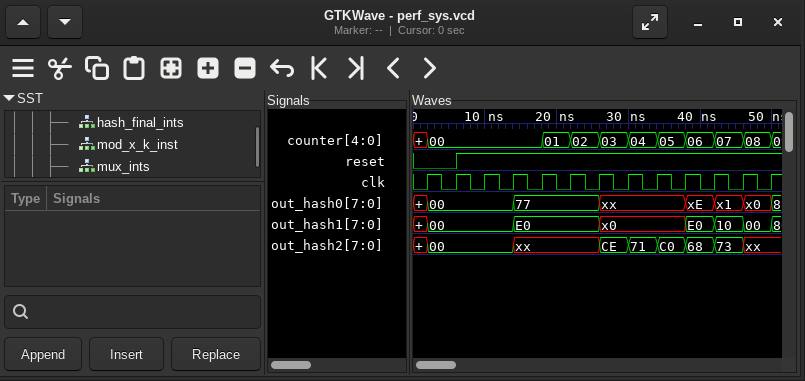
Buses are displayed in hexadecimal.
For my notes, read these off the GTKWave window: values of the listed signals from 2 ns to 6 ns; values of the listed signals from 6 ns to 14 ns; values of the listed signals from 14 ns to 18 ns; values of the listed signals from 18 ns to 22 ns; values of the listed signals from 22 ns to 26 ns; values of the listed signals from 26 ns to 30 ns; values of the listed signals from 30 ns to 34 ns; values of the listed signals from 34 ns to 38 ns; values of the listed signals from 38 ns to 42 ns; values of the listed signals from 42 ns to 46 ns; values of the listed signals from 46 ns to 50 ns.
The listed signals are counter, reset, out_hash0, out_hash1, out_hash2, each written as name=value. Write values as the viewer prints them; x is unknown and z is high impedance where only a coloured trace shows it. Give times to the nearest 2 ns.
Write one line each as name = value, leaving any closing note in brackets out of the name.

values of the listed signals from 2 ns to 6 ns = counter=00, reset=0, out_hash0=00, out_hash1=00, out_hash2=00
values of the listed signals from 6 ns to 14 ns = counter=00, reset=1, out_hash0=00, out_hash1=00, out_hash2=00
values of the listed signals from 14 ns to 18 ns = counter=00, reset=1, out_hash0=77, out_hash1=E0, out_hash2=xx
values of the listed signals from 18 ns to 22 ns = counter=01, reset=1, out_hash0=77, out_hash1=E0, out_hash2=xx
values of the listed signals from 22 ns to 26 ns = counter=02, reset=1, out_hash0=77, out_hash1=E0, out_hash2=xx
values of the listed signals from 26 ns to 30 ns = counter=03, reset=1, out_hash0=xx, out_hash1=x0, out_hash2=CE
values of the listed signals from 30 ns to 34 ns = counter=04, reset=1, out_hash0=xx, out_hash1=x0, out_hash2=71
values of the listed signals from 34 ns to 38 ns = counter=05, reset=1, out_hash0=xx, out_hash1=x0, out_hash2=C0
values of the listed signals from 38 ns to 42 ns = counter=06, reset=1, out_hash0=xE, out_hash1=E0, out_hash2=68
values of the listed signals from 42 ns to 46 ns = counter=07, reset=1, out_hash0=x1, out_hash1=10, out_hash2=73
values of the listed signals from 46 ns to 50 ns = counter=08, reset=1, out_hash0=x0, out_hash1=00, out_hash2=xx
